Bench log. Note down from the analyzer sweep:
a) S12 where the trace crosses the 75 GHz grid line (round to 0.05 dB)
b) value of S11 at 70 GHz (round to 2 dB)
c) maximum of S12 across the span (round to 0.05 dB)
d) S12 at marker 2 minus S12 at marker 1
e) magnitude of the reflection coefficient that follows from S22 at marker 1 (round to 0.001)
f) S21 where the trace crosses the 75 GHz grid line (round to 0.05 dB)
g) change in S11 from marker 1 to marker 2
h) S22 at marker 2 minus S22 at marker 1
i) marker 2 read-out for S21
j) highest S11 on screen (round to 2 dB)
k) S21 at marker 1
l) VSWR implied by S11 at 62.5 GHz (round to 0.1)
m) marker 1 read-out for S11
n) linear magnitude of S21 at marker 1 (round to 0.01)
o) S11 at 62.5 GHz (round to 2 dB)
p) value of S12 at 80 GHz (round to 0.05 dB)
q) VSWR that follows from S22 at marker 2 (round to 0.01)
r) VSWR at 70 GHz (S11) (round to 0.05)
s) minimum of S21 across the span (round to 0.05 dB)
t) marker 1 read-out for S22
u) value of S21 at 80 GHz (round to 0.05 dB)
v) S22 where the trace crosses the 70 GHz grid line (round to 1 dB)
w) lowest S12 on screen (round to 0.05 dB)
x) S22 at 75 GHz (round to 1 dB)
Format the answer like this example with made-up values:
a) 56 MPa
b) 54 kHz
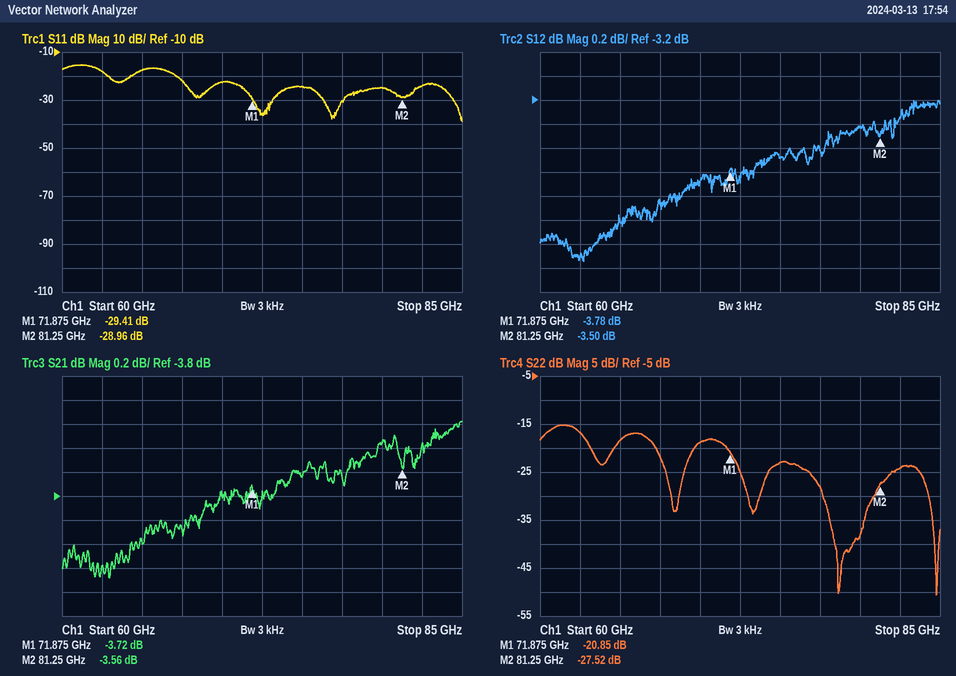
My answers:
a) -3.70 dB
b) -22 dB
c) -3.20 dB
d) 0.28 dB
e) 0.091
f) -3.65 dB
g) 0.45 dB
h) -6.67 dB
i) -3.56 dB
j) -16 dB
k) -3.72 dB
l) 1.3
m) -29.41 dB
n) 0.65
o) -18 dB
p) -3.40 dB
q) 1.09
r) 1.15
s) -4.50 dB
t) -20.85 dB
u) -3.35 dB
v) -19 dB
w) -4.55 dB
x) -23 dB
